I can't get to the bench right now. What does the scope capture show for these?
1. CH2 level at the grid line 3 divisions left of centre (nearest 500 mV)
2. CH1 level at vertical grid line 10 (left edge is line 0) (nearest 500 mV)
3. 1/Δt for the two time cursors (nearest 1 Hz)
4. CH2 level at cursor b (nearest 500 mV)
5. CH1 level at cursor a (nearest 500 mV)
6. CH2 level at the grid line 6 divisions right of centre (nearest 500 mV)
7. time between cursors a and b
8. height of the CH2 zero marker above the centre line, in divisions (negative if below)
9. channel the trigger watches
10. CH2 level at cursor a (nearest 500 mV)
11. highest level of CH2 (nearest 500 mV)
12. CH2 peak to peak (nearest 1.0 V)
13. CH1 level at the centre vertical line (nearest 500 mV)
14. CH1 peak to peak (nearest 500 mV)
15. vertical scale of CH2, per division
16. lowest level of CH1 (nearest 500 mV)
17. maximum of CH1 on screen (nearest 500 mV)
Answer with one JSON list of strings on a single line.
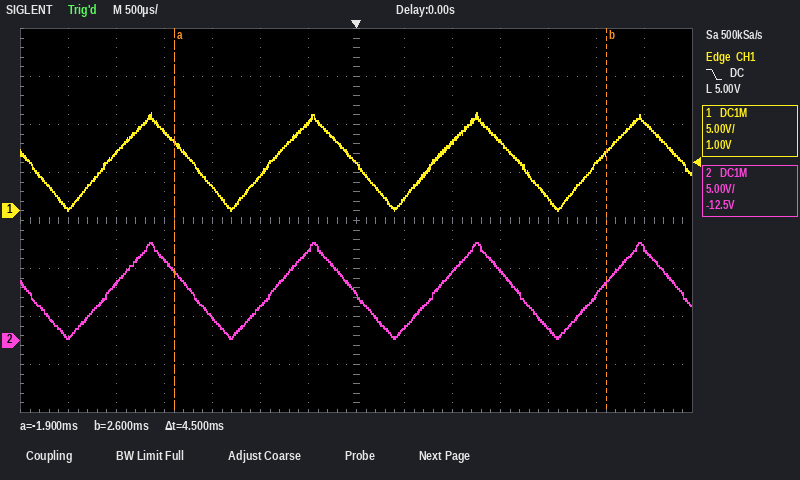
["2.5 V", "7.0 V", "222 Hz", "6.0 V", "7.0 V", "9.5 V", "4.5 ms", "-2.5 div", "CH1", "7.0 V", "10.0 V", "10.0 V", "5.0 V", "10.0 V", "5 V", "0.0 V", "10.0 V"]
